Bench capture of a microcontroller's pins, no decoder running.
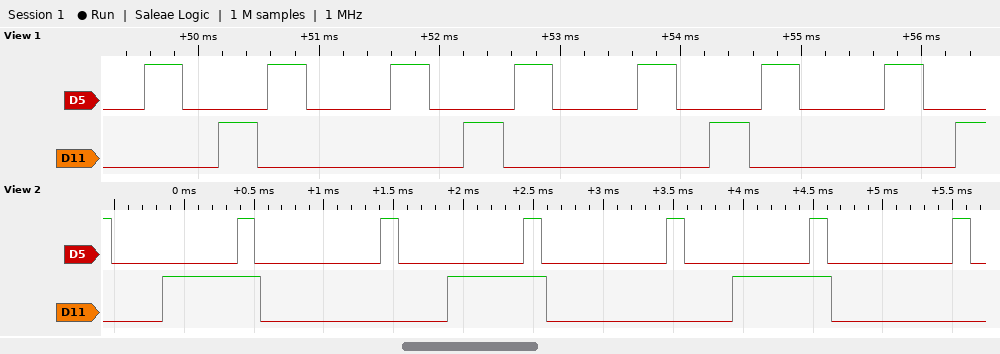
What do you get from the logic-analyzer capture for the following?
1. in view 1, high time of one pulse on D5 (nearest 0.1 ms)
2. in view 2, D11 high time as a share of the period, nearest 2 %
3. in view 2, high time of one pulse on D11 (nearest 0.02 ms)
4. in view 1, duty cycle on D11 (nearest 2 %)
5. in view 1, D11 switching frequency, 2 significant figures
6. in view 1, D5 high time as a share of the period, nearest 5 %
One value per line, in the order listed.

0.3 ms
34 %
0.70 ms
16 %
490 Hz
30 %
